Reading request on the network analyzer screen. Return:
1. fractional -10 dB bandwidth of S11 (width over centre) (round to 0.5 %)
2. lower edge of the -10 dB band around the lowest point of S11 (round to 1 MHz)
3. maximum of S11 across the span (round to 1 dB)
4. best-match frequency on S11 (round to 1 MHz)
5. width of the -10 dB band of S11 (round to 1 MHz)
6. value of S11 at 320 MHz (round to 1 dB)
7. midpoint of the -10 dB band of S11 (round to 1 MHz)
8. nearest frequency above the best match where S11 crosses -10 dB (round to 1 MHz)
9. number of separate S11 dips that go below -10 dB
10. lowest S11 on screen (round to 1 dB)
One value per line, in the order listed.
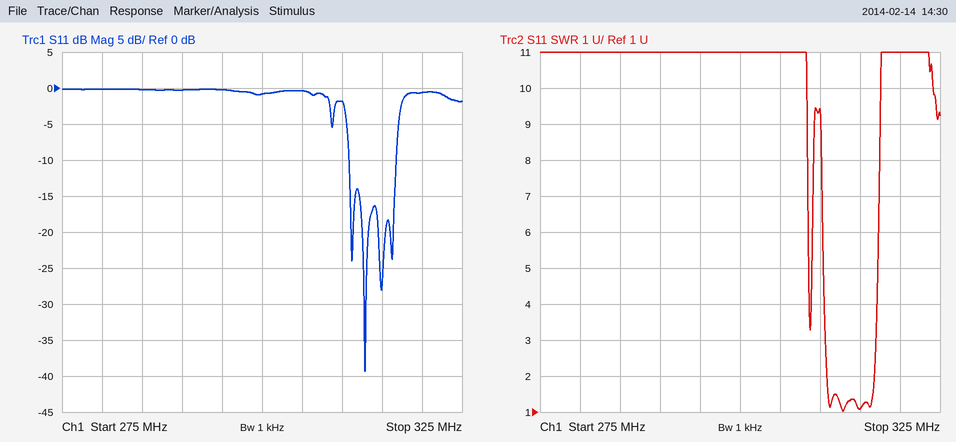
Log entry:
2.0 %
311 MHz
0 dB
313 MHz
6 MHz
-1 dB
314 MHz
317 MHz
4
-39 dB
